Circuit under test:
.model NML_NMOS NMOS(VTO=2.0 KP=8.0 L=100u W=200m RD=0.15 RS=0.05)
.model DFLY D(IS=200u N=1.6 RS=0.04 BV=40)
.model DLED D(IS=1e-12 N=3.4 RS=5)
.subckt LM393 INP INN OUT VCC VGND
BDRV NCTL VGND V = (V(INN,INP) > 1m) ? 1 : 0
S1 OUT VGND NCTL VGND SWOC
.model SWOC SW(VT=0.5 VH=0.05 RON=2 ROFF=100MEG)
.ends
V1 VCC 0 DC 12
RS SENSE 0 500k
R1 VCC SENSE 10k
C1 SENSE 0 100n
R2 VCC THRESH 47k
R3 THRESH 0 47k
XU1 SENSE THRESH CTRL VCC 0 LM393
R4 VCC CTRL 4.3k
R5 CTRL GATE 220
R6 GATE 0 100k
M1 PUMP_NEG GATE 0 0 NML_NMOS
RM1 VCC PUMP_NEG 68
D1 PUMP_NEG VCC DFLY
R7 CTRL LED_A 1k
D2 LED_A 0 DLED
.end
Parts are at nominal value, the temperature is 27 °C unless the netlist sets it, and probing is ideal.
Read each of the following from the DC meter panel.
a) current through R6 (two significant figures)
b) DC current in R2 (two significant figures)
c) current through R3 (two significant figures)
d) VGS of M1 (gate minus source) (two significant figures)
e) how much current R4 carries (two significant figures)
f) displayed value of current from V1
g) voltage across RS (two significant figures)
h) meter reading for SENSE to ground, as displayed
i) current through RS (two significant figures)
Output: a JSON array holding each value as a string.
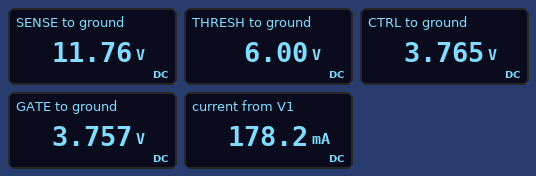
["38 µA", "130 µA", "130 µA", "3.8 V", "1.9 mA", "178.2 mA", "12 V", "11.76 V", "24 µA"]
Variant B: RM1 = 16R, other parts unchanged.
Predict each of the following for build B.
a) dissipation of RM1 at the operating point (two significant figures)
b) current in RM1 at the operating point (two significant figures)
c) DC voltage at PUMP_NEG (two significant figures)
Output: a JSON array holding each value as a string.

["8.8 W", "740 mA", "150 mV"]
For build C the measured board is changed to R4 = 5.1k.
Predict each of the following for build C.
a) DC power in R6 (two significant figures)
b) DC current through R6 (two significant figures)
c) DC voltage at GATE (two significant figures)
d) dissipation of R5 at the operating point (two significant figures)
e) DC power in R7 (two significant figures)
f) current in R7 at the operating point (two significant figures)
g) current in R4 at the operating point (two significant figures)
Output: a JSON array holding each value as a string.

["120 µW", "35 µA", "3.5 V", "270 nW", "2.7 mW", "1.6 mA", "1.7 mA"]
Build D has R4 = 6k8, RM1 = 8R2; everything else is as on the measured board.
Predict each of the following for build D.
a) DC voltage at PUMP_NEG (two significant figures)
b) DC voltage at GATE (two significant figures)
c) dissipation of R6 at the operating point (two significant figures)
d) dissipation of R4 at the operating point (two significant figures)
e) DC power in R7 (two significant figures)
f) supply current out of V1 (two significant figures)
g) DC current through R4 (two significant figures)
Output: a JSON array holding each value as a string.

["290 mV", "3.1 V", "97 µW", "12 mW", "1.6 mW", "1.4 A", "1.3 mA"]
